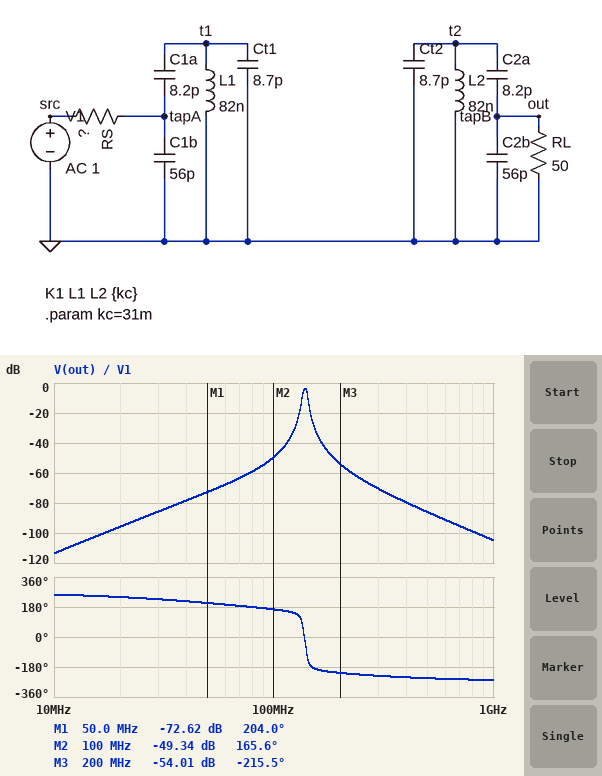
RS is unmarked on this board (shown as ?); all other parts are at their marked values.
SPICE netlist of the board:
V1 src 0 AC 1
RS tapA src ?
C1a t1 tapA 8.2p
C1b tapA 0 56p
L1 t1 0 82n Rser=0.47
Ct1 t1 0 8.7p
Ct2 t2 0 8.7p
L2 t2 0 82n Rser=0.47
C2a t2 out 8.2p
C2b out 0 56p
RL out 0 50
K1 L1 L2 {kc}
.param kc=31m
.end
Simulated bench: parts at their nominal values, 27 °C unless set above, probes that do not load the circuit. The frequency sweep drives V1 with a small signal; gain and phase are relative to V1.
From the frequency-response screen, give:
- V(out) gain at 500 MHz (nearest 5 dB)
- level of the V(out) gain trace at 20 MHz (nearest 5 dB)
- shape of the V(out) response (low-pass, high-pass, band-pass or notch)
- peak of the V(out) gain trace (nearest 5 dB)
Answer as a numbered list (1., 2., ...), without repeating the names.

1. -85 dB
2. -95 dB
3. band-pass
4. -5 dB
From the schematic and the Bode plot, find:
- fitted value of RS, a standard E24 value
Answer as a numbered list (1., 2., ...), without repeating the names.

1. 18 Ω
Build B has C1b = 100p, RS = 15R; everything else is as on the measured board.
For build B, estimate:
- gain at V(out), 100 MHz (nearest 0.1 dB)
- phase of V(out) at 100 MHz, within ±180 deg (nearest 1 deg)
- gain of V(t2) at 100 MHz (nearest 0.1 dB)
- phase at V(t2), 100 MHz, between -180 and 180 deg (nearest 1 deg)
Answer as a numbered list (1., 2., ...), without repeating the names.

1. -50.6 dB
2. 157 deg
3. -31.7 dB
4. 130 deg
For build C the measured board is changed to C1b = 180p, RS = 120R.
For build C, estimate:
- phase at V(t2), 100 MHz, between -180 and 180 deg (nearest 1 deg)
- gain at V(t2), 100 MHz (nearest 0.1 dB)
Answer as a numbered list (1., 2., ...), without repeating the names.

1. 91 deg
2. -51.7 dB
